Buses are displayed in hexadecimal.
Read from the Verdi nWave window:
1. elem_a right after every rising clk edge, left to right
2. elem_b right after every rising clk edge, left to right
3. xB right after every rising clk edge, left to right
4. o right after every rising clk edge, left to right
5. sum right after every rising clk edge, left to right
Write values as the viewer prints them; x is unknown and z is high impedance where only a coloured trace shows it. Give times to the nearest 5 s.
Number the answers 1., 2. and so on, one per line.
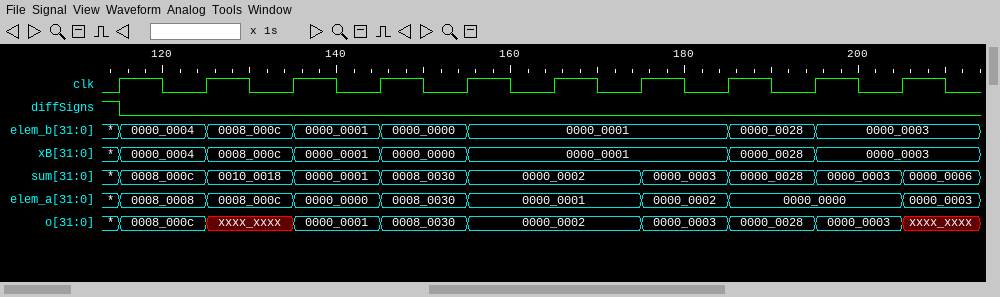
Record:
1. 0008_0008, 0008_000c, 0000_0000, 0008_0030, 0000_0001, 0000_0001, 0000_0002, 0000_0000, 0000_0000, 0000_0003
2. 0000_0004, 0008_000c, 0000_0001, 0000_0000, 0000_0001, 0000_0001, 0000_0001, 0000_0028, 0000_0003, 0000_0003
3. 0000_0004, 0008_000c, 0000_0001, 0000_0000, 0000_0001, 0000_0001, 0000_0001, 0000_0028, 0000_0003, 0000_0003
4. 0008_000c, xxxx_xxxx, 0000_0001, 0008_0030, 0000_0002, 0000_0002, 0000_0003, 0000_0028, 0000_0003, xxxx_xxxx
5. 0008_000c, 0010_0018, 0000_0001, 0008_0030, 0000_0002, 0000_0002, 0000_0003, 0000_0028, 0000_0003, 0000_0006
